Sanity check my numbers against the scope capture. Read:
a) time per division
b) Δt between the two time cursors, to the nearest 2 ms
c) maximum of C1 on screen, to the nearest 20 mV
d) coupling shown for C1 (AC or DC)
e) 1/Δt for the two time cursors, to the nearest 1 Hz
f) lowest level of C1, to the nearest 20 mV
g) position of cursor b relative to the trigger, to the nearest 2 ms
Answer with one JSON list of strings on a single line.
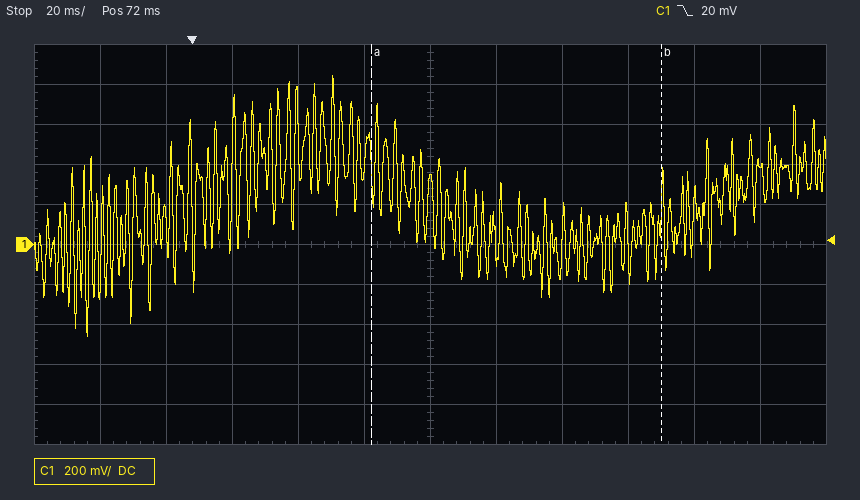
["20 ms", "88 ms", "840 mV", "DC", "11 Hz", "-460 mV", "+142 ms"]
